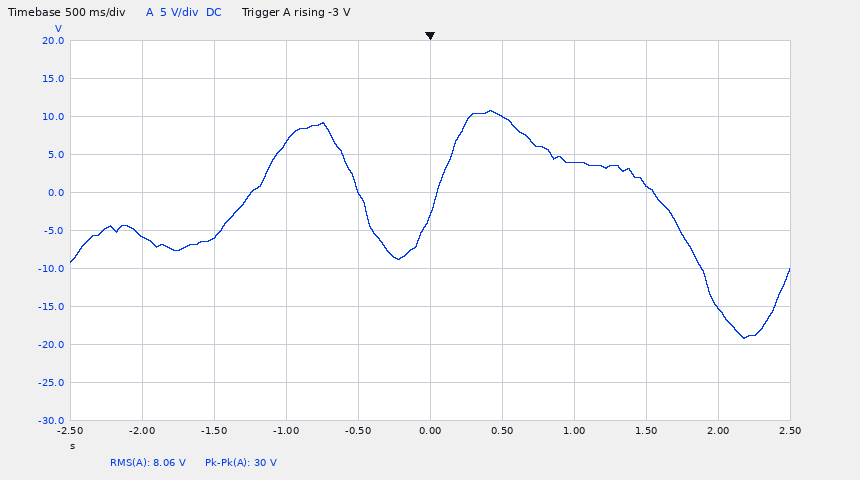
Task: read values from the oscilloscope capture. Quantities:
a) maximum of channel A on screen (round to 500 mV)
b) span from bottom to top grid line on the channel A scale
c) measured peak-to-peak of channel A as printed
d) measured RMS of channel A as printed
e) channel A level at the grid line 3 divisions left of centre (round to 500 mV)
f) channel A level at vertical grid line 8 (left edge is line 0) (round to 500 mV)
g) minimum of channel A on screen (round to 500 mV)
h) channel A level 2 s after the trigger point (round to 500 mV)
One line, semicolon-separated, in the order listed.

11.0 V; 50 V; 30 V; 8.06 V; -6.0 V; 1.0 V; -19.0 V; -15.0 V
